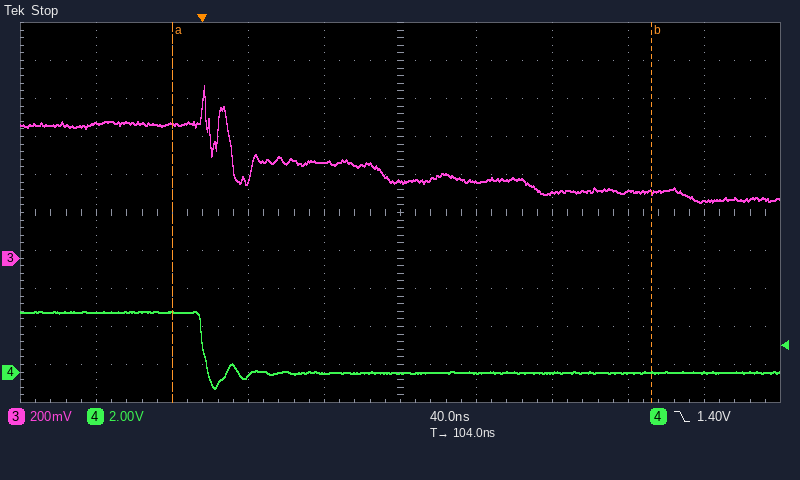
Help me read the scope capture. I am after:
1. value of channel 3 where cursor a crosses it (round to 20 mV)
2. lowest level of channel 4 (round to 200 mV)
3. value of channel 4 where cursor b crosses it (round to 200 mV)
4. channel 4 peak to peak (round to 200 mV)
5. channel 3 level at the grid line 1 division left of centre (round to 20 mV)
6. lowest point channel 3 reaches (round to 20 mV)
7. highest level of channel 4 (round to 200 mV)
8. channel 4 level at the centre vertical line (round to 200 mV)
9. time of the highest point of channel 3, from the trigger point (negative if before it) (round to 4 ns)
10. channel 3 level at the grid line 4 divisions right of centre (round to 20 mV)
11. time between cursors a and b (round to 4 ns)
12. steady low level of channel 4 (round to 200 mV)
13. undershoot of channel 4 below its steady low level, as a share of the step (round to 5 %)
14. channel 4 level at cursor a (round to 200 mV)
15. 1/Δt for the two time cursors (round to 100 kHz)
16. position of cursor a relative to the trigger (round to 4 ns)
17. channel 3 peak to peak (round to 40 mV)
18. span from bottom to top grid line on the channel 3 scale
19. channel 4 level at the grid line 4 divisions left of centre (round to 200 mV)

700 mV
-800 mV
0.0 V
4.0 V
500 mV
300 mV
3.2 V
0.0 V
0 ns
300 mV
252 ns
0.0 V
25 %
3.2 V
4.0 MHz
-16 ns
600 mV
2 V
3.2 V
